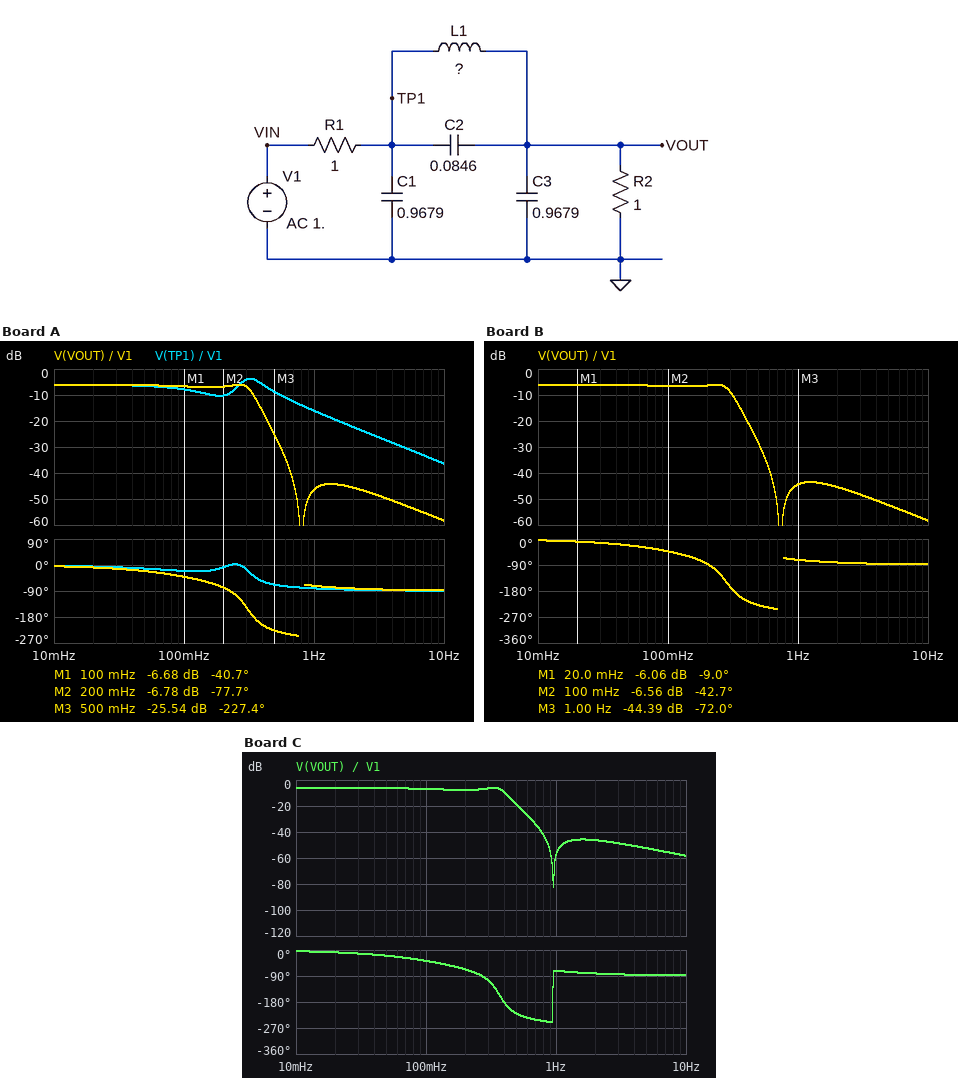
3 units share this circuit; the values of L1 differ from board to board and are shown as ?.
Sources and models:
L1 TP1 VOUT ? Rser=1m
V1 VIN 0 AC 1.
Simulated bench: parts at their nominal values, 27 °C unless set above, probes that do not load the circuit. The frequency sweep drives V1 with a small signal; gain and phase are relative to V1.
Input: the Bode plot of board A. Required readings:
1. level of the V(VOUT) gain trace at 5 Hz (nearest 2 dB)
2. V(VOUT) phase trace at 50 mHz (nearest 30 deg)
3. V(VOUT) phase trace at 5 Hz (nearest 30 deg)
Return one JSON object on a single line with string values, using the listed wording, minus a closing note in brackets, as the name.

{"level of the V(VOUT) gain trace at 5 Hz": "-52 dB", "V(VOUT) phase trace at 50 mHz": "-30 deg", "V(VOUT) phase trace at 5 Hz": "-90 deg"}
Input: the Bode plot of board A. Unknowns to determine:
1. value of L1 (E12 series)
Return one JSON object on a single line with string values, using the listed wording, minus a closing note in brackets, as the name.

{"value of L1": "470 mH"}
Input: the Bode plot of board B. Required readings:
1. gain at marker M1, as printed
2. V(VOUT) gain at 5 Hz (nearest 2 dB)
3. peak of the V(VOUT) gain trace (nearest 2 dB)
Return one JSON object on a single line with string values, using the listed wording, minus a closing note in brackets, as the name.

{"gain at marker M1, as printed": "-6.06 dB", "V(VOUT) gain at 5 Hz": "-52 dB", "peak of the V(VOUT) gain trace": "-6 dB"}
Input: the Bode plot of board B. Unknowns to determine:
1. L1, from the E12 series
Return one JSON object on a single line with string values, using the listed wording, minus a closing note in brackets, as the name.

{"L1, from the E12 series": "560 mH"}
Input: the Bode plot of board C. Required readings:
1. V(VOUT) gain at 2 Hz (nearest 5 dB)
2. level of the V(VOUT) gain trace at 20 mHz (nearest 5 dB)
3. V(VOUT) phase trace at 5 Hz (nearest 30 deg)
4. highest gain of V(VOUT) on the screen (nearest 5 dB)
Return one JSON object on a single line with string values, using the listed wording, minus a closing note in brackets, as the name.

{"V(VOUT) gain at 2 Hz": "-45 dB", "level of the V(VOUT) gain trace at 20 mHz": "-5 dB", "V(VOUT) phase trace at 5 Hz": "-90 deg", "highest gain of V(VOUT) on the screen": "-5 dB"}
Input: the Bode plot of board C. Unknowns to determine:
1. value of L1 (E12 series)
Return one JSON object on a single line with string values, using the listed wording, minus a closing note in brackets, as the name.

{"value of L1": "330 mH"}
